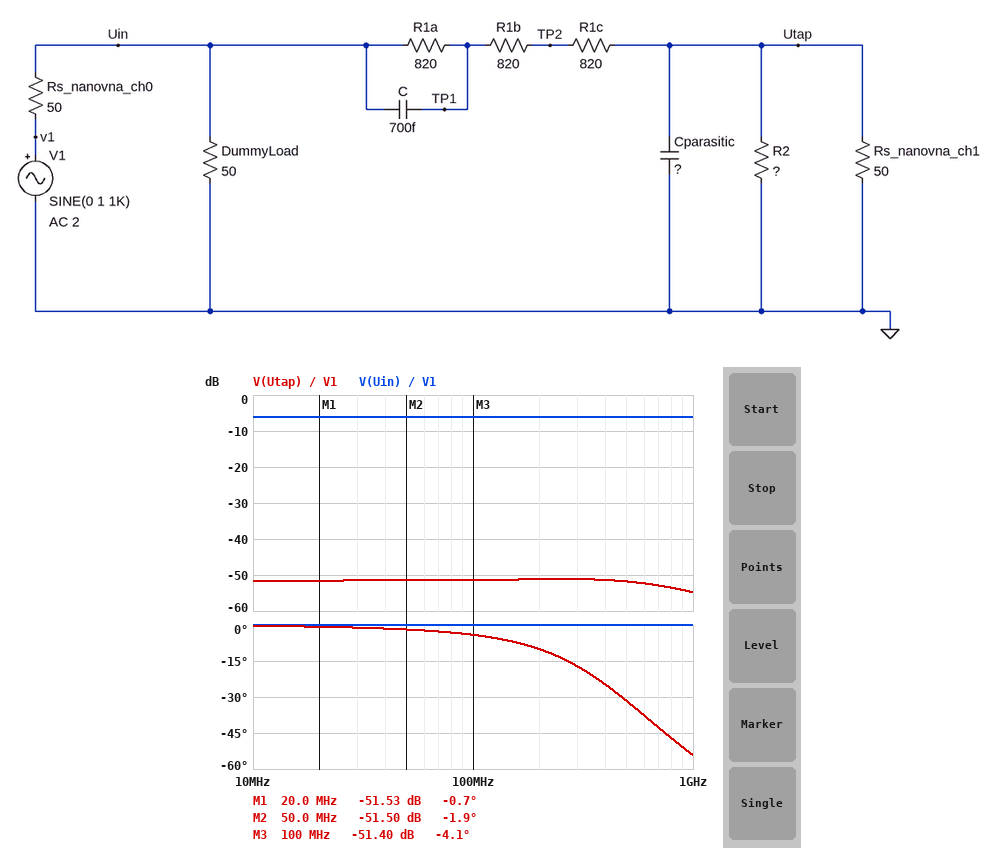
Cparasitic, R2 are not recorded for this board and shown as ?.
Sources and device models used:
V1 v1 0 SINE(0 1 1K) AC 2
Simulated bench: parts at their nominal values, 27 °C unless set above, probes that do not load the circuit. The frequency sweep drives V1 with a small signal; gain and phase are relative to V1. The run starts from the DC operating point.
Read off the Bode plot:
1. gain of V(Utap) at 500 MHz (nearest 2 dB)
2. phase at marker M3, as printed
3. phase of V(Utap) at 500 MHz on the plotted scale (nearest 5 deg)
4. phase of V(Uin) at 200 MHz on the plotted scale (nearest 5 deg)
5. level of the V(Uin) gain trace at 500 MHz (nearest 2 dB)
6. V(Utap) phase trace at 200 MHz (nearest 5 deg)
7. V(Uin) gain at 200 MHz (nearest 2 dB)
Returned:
-52 dB
-4.1 deg
-30 deg
0 deg
-6 dB
-10 deg
-6 dB
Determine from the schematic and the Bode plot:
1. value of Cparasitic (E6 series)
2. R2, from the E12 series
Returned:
22 pF
18 Ω
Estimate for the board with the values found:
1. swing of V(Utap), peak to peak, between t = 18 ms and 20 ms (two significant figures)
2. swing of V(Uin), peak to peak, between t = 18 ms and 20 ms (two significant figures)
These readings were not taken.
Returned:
5.3 mV
990 mV
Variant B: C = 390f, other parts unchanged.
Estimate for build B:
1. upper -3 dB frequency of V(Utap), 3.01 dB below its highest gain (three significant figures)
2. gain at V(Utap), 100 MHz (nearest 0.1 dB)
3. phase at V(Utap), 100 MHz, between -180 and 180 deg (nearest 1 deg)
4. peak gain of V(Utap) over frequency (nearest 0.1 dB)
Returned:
848 MHz
-51.6 dB
-7 deg
-51.5 dB
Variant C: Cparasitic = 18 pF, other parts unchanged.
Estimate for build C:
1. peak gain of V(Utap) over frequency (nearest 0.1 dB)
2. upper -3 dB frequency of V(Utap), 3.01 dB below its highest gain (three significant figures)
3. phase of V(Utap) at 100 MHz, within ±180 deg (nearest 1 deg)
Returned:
-50.8 dB
1.06 GHz
-2 deg
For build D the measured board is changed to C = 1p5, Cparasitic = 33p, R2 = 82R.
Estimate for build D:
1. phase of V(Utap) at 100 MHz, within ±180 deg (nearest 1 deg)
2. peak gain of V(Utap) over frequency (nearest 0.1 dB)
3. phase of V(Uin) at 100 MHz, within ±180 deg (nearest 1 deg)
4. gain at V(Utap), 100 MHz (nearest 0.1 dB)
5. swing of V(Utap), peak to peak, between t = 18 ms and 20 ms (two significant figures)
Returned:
-22 deg
-44.2 dB
0 deg
-44.7 dB
12 mV
